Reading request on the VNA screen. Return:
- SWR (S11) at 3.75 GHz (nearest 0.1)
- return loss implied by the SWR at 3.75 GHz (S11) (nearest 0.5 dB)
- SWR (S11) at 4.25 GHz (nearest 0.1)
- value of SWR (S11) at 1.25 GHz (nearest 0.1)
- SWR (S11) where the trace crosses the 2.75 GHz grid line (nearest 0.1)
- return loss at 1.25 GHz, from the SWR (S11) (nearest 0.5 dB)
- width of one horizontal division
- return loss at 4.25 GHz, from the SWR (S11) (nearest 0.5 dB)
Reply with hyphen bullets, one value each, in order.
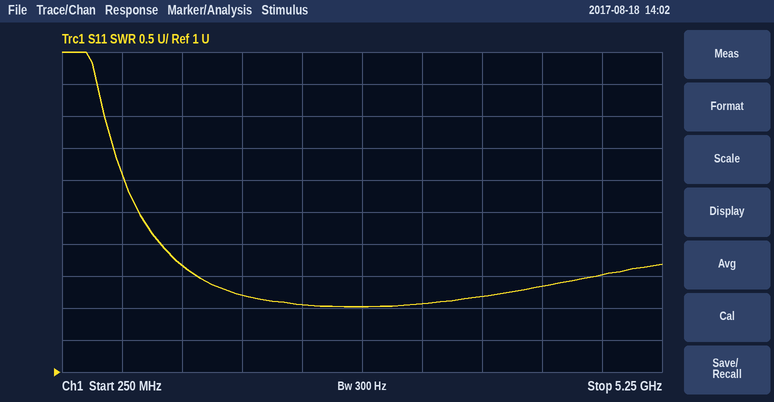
- 2.2
- 8.5 dB
- 2.3
- 2.7
- 2.0
- 7.0 dB
- 500 MHz
- 8.0 dB
